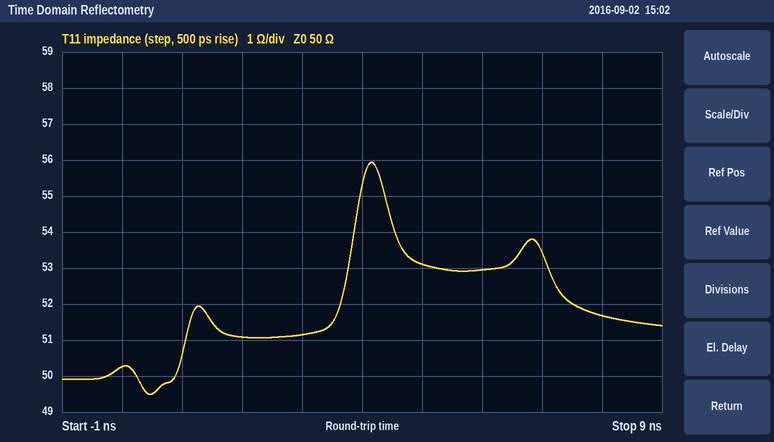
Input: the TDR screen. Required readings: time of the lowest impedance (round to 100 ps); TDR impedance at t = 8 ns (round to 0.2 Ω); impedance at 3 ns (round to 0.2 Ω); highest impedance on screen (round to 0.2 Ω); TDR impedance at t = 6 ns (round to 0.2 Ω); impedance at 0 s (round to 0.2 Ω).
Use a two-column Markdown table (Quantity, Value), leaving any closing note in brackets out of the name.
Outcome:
| Quantity | Value |
|---|---|
| time of the lowest impedance | 500 ps |
| TDR impedance at t = 8 ns | 51.6 Ω |
| impedance at 3 ns | 51.2 Ω |
| highest impedance on screen | 56.0 Ω |
| TDR impedance at t = 6 ns | 53.0 Ω |
| impedance at 0 s | 50.2 Ω |
